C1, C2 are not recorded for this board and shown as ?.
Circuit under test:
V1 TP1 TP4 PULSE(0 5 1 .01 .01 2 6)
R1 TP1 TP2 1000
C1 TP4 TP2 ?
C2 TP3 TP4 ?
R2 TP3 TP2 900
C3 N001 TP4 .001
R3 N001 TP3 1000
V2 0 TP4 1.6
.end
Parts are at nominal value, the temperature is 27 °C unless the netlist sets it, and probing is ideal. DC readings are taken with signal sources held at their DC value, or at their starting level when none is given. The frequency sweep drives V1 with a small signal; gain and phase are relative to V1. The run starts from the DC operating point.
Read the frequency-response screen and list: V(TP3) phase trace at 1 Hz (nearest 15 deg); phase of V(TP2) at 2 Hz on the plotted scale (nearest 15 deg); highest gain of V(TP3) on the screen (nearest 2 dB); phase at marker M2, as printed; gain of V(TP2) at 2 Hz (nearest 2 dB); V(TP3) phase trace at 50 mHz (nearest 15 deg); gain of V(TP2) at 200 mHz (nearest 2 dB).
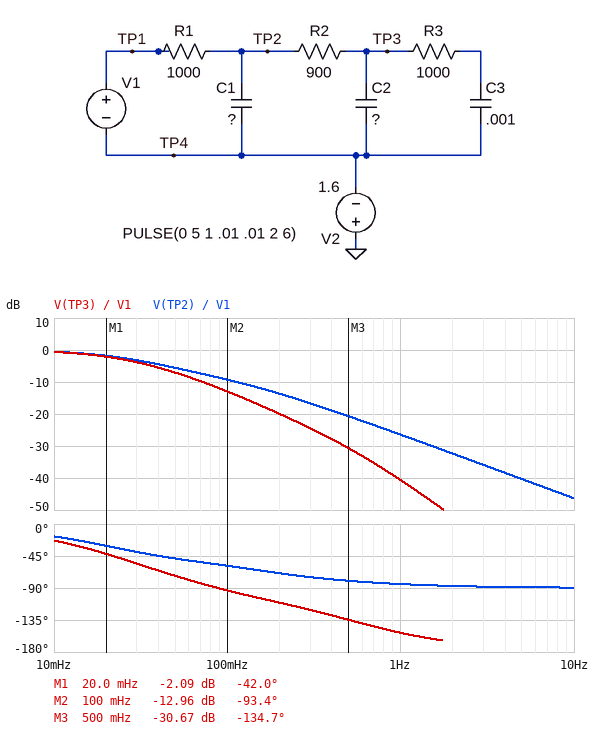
-150 deg
-90 deg
0 dB
-93.4 deg
-32 dB
-75 deg
-14 dB
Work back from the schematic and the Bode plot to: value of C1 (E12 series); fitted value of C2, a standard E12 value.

3.3 mF
820 µF
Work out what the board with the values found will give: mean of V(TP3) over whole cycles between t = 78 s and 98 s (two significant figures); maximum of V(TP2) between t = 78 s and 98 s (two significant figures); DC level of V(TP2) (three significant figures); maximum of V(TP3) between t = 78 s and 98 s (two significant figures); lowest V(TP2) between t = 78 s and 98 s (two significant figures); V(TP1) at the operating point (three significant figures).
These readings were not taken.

75 mV
1.0 V
-1.60 V
460 mV
-640 mV
-1.60 V
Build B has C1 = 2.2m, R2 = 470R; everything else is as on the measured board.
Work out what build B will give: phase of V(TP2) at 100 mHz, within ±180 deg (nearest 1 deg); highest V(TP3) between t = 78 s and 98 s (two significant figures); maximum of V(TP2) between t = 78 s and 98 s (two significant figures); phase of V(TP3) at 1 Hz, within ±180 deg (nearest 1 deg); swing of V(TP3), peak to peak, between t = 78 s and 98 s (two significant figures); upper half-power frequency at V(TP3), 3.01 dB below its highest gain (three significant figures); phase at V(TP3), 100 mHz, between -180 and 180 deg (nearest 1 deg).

-53 deg
790 mV
1.2 V
-139 deg
1.3 V
33.4 mHz
-75 deg
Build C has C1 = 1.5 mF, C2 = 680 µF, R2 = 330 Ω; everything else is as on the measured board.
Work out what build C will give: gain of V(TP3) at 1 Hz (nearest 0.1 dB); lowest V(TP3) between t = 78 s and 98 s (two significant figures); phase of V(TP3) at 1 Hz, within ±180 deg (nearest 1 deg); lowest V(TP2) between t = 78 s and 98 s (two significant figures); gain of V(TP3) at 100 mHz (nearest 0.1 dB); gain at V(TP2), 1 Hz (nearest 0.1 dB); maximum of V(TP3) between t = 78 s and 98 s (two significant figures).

-26.7 dB
-740 mV
-122 deg
-880 mV
-7.8 dB
-20.8 dB
1.1 V
